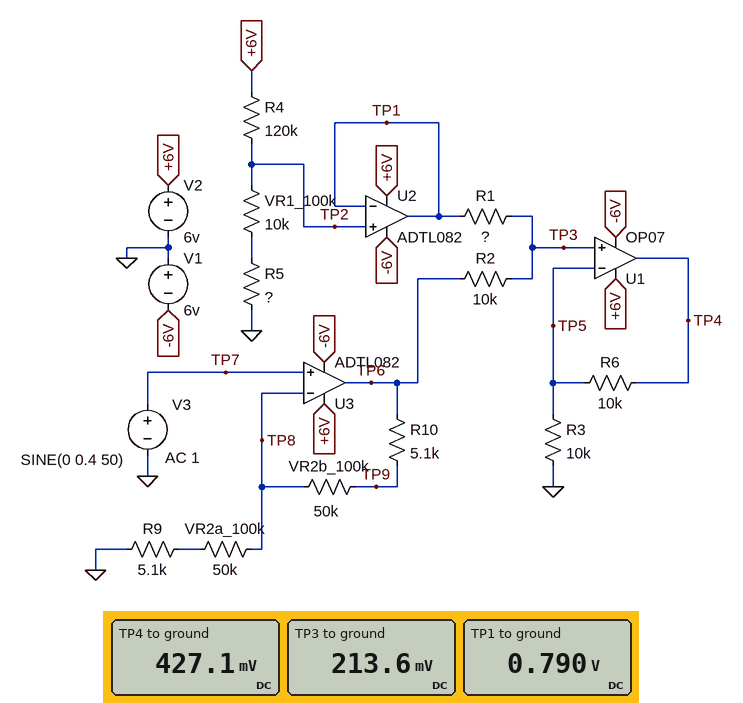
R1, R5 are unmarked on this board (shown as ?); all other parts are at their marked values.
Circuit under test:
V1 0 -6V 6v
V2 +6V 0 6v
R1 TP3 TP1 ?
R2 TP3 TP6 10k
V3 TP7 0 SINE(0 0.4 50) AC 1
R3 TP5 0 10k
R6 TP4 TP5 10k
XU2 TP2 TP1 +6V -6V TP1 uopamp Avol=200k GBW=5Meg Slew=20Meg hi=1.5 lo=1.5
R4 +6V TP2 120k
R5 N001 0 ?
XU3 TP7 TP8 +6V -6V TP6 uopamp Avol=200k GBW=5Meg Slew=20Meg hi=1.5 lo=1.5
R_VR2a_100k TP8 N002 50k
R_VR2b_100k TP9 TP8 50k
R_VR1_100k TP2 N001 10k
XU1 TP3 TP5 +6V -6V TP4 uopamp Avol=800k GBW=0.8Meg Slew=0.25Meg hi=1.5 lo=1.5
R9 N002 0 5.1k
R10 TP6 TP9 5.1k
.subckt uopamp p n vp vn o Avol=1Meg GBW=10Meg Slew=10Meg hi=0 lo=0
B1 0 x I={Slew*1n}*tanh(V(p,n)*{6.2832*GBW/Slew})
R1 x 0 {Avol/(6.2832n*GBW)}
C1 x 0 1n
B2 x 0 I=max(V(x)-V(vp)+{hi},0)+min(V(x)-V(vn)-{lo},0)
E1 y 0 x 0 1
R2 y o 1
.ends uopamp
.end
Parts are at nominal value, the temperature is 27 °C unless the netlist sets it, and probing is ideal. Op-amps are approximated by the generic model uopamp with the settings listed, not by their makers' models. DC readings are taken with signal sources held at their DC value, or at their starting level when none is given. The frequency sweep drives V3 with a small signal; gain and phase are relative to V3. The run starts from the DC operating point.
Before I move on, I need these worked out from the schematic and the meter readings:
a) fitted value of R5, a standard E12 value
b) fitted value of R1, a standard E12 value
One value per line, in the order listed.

8.2 kΩ
27 kΩ
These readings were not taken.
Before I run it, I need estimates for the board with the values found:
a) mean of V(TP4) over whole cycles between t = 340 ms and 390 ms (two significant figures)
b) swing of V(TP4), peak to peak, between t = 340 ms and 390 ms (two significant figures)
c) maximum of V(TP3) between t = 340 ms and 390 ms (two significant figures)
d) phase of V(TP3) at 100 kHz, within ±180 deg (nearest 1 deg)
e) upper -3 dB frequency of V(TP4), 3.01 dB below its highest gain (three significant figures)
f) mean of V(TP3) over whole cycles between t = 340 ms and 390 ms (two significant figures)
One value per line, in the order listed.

430 mV
2.3 V
800 mV
-2 deg
390 kHz
210 mV
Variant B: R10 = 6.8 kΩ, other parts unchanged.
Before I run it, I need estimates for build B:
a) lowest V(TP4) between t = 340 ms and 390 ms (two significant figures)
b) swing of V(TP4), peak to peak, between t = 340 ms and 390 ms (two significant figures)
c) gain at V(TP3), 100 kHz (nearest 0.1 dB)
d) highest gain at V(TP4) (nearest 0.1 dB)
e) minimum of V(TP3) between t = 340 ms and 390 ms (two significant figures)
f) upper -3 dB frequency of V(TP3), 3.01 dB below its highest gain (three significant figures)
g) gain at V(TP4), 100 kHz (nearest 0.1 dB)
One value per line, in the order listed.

-760 mV
2.4 V
3.4 dB
9.4 dB
-380 mV
2.46 MHz
9.2 dB
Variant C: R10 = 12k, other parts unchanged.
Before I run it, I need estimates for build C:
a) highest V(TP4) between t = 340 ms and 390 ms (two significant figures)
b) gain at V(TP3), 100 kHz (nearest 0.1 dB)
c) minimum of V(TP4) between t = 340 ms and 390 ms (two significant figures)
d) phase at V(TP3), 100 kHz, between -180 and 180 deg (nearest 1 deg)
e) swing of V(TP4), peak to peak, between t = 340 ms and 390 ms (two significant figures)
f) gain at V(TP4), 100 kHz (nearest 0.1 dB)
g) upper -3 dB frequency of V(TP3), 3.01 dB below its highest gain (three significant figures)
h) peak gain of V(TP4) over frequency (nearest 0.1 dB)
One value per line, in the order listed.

1.7 V
3.8 dB
-810 mV
-2 deg
2.5 V
9.6 dB
2.35 MHz
9.8 dB
